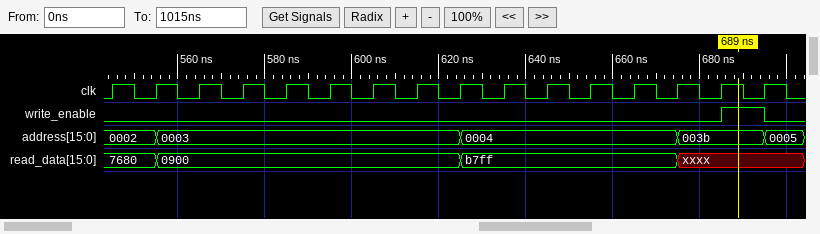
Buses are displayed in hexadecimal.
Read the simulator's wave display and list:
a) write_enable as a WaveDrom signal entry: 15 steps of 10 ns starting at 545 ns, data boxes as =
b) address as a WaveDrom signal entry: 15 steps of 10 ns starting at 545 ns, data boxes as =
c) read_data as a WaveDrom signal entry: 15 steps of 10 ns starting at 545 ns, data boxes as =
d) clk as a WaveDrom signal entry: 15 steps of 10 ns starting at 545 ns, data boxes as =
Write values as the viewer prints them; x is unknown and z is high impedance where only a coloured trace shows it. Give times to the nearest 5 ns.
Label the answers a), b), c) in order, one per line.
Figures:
a) {name: 'write_enable', wave: '0.............1'}
b) {name: 'address', wave: '==......=....=.', data: '0002 0003 0004 003b'}
c) {name: 'read_data', wave: '==......=....x.', data: '7680 0900 b7ff'}
d) {name: 'clk', wave: 'p..............'}
